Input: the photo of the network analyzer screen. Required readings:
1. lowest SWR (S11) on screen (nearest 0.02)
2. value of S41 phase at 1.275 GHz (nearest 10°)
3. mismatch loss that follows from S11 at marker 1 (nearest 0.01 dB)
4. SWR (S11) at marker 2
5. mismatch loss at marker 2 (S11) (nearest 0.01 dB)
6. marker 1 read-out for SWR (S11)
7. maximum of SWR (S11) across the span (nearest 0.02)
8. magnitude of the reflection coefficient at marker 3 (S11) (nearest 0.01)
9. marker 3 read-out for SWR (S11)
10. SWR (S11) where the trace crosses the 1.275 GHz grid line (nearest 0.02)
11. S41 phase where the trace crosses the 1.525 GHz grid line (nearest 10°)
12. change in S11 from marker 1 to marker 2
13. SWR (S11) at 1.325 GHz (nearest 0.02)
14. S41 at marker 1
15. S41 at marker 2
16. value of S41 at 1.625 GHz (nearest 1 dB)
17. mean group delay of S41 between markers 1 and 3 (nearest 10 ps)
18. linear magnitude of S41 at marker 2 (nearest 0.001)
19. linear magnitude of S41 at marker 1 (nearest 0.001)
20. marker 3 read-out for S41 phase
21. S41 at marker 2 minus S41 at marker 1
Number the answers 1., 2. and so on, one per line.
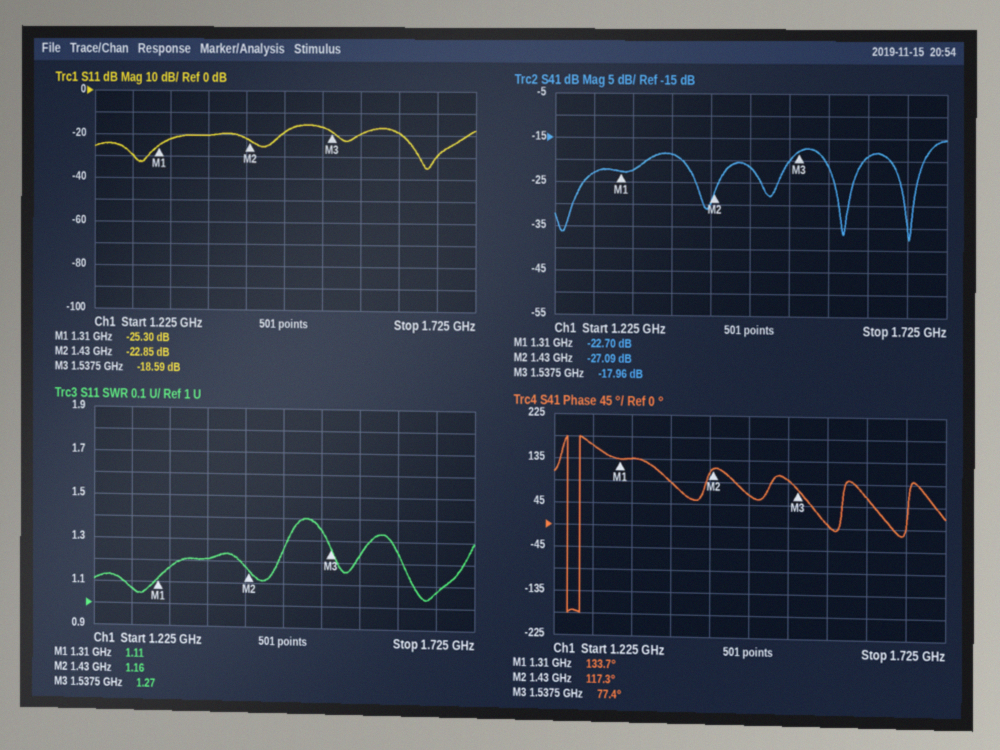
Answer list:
1. 1.04
2. 160°
3. 0.01 dB
4. 1.16
5. 0.02 dB
6. 1.11
7. 1.40
8. 0.12
9. 1.27
10. 1.06
11. 100°
12. 2.45 dB
13. 1.16
14. -22.70 dB
15. -27.09 dB
16. -19 dB
17. 690 ps
18. 0.044
19. 0.073
20. 77.4°
21. -4.39 dB
